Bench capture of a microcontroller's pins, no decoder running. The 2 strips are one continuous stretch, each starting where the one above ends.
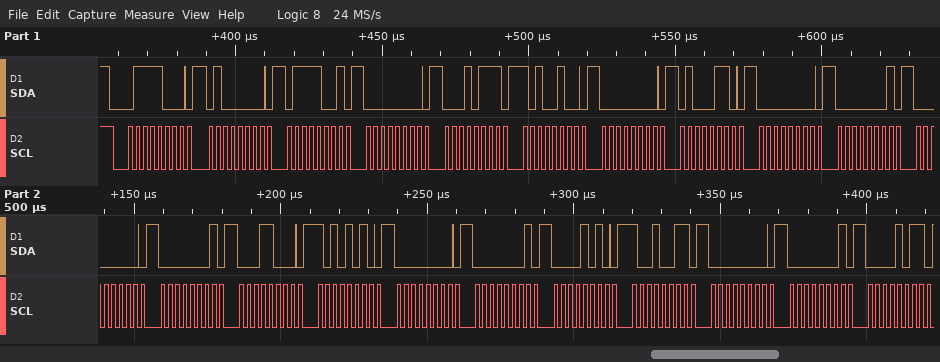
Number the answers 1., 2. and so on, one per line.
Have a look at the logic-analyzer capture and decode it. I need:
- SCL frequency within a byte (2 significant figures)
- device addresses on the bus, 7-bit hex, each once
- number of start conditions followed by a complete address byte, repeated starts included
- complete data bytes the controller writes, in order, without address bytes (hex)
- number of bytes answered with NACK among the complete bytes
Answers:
1. 400 kHz
2. 0x3C
3. 1
4. 40 79 00 17 A4 00 46 00 01 00 01 18 AA 00 01 0A 93 00 01 0B
5. 0
